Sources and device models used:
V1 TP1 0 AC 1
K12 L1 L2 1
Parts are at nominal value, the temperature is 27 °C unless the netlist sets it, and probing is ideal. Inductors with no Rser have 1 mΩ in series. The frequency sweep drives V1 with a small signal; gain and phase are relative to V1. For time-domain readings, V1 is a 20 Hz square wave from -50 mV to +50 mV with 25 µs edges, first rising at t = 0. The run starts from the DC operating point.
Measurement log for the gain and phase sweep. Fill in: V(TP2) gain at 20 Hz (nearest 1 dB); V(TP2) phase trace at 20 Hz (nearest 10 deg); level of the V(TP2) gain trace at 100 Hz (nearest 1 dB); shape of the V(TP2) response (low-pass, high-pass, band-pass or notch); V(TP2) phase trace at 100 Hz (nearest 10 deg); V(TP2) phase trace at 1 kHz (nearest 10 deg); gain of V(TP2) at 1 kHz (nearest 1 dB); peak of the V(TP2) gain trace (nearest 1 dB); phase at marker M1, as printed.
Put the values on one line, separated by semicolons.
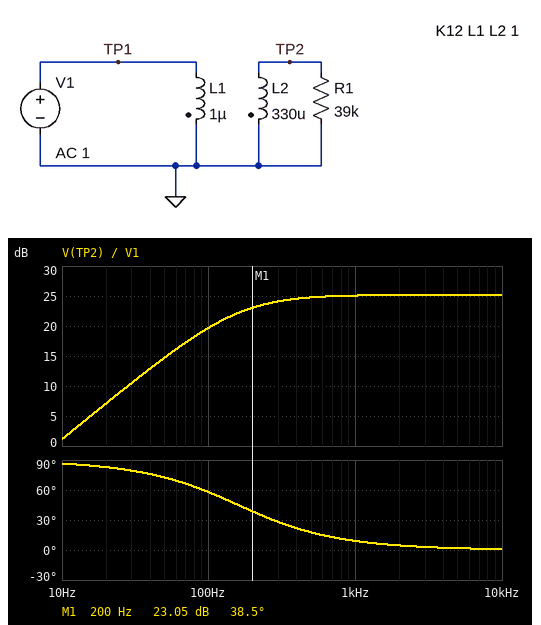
7 dB; 80 deg; 20 dB; high-pass; 60 deg; 10 deg; 25 dB; 25 dB; 38.5 deg
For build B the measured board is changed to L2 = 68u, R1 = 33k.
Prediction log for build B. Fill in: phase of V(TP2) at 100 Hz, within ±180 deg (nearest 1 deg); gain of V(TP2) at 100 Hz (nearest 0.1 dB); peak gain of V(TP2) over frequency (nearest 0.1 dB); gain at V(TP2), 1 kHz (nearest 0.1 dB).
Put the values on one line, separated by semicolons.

58 deg; 12.8 dB; 18.3 dB; 18.2 dB
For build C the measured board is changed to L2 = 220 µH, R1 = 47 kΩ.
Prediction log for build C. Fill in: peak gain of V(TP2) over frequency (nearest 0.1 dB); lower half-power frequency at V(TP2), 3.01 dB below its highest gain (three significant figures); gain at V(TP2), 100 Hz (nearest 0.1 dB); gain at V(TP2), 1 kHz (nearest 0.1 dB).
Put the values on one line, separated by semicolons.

23.4 dB; 159 Hz; 17.9 dB; 23.3 dB
